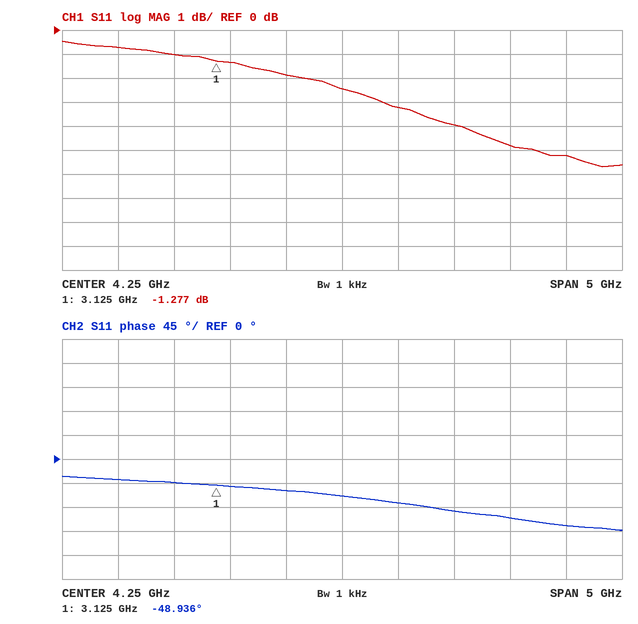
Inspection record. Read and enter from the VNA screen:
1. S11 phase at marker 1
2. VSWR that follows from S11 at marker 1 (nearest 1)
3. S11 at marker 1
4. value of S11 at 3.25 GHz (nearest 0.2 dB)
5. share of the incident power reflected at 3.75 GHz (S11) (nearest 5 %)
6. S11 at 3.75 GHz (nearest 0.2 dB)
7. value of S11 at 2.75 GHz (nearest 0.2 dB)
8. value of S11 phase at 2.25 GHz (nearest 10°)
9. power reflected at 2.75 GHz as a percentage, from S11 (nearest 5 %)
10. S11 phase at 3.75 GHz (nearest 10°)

-48.936°
14
-1.277 dB
-1.4 dB
65 %
-1.8 dB
-1.0 dB
-40°
80 %
-60°
